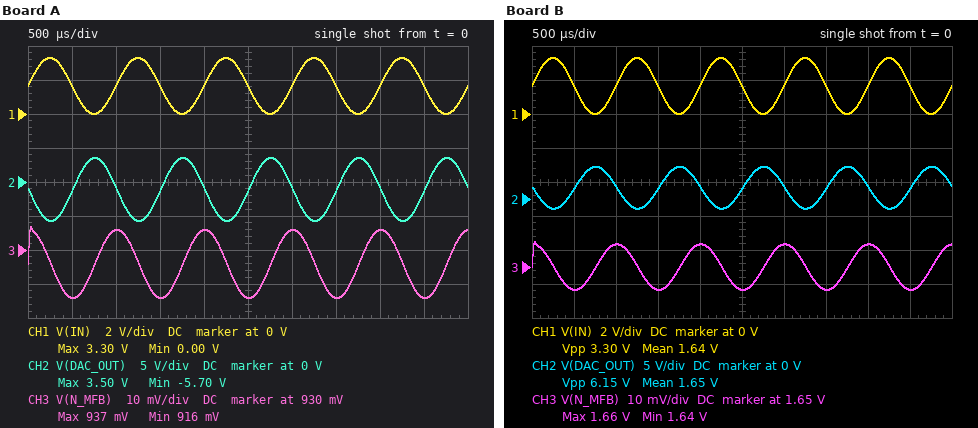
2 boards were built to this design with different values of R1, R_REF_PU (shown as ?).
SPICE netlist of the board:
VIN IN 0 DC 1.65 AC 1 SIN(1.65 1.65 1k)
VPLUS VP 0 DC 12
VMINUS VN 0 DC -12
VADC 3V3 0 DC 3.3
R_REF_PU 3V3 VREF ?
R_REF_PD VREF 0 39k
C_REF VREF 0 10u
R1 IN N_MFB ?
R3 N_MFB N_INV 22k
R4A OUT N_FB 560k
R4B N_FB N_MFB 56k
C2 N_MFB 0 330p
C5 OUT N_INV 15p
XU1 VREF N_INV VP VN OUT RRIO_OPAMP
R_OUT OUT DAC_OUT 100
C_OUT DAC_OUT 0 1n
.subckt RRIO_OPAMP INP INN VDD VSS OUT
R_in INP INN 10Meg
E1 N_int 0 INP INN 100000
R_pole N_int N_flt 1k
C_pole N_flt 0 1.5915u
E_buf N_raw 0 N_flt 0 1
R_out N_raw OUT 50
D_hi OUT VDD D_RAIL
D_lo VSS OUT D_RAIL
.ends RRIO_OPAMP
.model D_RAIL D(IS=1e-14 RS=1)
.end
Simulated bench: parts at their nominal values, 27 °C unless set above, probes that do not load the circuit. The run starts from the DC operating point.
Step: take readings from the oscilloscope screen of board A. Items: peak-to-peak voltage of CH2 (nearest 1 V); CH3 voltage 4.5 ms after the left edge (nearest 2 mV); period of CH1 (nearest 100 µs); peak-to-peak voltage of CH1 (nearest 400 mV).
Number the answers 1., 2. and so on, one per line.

1. 9 V
2. 916 mV
3. 1.0 ms
4. 3.2 V
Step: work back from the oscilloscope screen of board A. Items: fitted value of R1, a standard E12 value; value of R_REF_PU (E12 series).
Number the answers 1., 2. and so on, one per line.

1. 220 kΩ
2. 100 kΩ
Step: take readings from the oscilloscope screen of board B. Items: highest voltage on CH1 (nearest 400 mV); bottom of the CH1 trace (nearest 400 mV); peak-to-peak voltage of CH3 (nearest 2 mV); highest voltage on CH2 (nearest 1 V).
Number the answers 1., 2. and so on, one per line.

1. 3.2 V
2. 0 V
3. 14 mV
4. 5 V
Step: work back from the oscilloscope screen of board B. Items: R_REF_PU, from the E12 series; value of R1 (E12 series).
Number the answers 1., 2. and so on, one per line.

1. 39 kΩ
2. 330 kΩ
